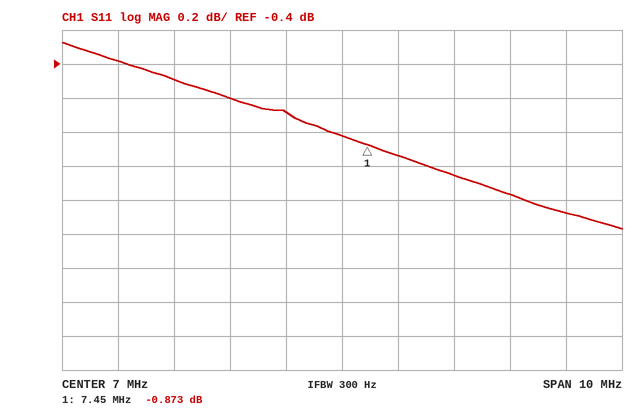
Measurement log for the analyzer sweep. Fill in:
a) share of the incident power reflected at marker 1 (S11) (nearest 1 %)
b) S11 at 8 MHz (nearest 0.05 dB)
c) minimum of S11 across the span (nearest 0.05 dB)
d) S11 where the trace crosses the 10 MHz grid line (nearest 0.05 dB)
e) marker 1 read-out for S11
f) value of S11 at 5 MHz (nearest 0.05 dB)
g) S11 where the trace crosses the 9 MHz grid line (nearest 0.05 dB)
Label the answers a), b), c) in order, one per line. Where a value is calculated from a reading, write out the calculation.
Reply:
a) 10^(-0.873/10) ≈ 82 %
b) -0.95 dB
c) -1.35 dB
d) -1.15 dB
e) -0.873 dB
f) -0.60 dB
g) -1.05 dB
